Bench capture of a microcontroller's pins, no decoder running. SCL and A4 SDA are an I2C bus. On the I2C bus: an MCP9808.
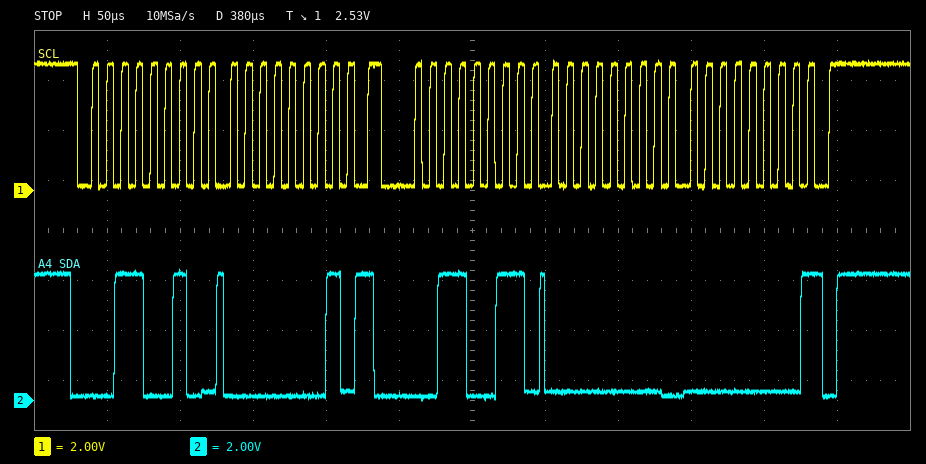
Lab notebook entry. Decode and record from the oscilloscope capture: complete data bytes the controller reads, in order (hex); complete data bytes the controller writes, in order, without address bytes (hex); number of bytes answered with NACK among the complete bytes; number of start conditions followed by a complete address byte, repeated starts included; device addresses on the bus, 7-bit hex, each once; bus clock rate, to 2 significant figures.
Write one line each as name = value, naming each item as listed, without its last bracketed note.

complete data bytes the controller reads, in order = 00 00
complete data bytes the controller writes, in order, without address bytes = 01
number of bytes answered with NACK among the complete bytes = 1
number of start conditions followed by a complete address byte, repeated starts included = 2
device addresses on the bus, 7-bit hex, each once = 0x19
bus clock rate, to 2 significant figures = 100 kHz
